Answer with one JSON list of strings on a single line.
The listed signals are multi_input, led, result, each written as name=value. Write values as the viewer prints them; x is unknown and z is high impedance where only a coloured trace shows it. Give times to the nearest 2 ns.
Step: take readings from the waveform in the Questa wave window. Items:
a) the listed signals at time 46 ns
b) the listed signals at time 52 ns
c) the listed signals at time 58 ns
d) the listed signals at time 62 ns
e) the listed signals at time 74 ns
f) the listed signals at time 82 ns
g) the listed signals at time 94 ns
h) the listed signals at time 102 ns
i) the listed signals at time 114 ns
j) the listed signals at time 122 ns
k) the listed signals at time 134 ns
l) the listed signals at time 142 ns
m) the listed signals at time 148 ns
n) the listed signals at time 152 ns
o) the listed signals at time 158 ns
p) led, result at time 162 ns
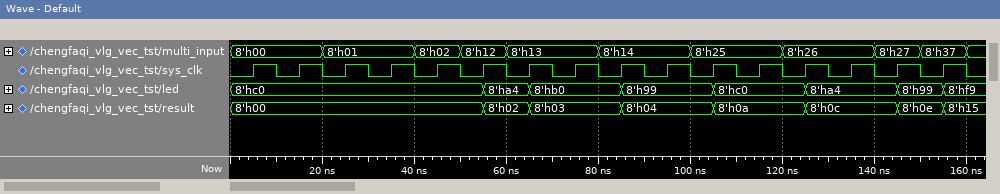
["multi_input=8'h02, led=8'hc0, result=8'h00", "multi_input=8'h12, led=8'hc0, result=8'h00", "multi_input=8'h12, led=8'ha4, result=8'h02", "multi_input=8'h13, led=8'ha4, result=8'h02", "multi_input=8'h13, led=8'hb0, result=8'h03", "multi_input=8'h14, led=8'hb0, result=8'h03", "multi_input=8'h14, led=8'h99, result=8'h04", "multi_input=8'h25, led=8'h99, result=8'h04", "multi_input=8'h25, led=8'hc0, result=8'h0a", "multi_input=8'h26, led=8'hc0, result=8'h0a", "multi_input=8'h26, led=8'ha4, result=8'h0c", "multi_input=8'h27, led=8'ha4, result=8'h0c", "multi_input=8'h27, led=8'h99, result=8'h0e", "multi_input=8'h37, led=8'h99, result=8'h0e", "multi_input=8'h37, led=8'hf9, result=8'h15", "led=8'hf9, result=8'h15"]
